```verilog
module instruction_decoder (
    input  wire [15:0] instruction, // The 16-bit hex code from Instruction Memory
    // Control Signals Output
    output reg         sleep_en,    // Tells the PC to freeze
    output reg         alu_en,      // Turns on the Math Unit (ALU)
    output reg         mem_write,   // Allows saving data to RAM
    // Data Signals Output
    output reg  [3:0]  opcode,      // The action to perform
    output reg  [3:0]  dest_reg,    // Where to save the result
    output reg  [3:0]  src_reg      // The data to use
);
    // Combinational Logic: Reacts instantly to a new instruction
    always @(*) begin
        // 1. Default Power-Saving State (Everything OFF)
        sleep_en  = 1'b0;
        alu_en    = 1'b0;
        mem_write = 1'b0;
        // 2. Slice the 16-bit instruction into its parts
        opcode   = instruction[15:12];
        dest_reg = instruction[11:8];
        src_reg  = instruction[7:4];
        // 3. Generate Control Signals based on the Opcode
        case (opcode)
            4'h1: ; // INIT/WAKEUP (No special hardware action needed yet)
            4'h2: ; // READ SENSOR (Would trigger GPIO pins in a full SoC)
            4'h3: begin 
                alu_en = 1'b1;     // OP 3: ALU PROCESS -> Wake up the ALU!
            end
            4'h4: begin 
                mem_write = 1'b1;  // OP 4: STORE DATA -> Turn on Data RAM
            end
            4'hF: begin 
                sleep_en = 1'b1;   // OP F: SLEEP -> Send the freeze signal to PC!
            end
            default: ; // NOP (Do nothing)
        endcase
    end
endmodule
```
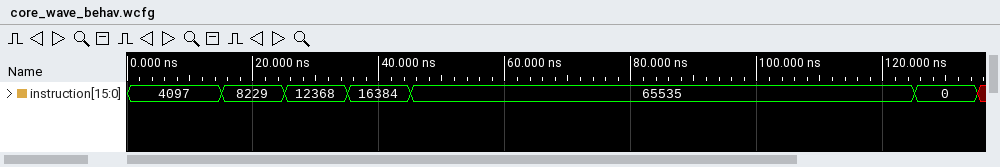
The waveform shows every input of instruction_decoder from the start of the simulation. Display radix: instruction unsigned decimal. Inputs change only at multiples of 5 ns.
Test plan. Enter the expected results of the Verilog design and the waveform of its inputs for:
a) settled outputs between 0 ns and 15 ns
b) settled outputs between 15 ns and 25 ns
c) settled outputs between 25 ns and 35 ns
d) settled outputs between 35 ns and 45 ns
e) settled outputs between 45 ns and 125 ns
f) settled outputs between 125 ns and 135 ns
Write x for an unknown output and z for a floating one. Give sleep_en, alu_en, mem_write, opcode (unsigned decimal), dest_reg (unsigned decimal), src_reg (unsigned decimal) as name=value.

sleep_en=0, alu_en=0, mem_write=0, opcode=1, dest_reg=0, src_reg=0
sleep_en=0, alu_en=0, mem_write=0, opcode=2, dest_reg=0, src_reg=2
sleep_en=0, alu_en=1, mem_write=0, opcode=3, dest_reg=0, src_reg=5
sleep_en=0, alu_en=0, mem_write=1, opcode=4, dest_reg=0, src_reg=0
sleep_en=1, alu_en=0, mem_write=0, opcode=15, dest_reg=15, src_reg=15
sleep_en=0, alu_en=0, mem_write=0, opcode=0, dest_reg=0, src_reg=0
